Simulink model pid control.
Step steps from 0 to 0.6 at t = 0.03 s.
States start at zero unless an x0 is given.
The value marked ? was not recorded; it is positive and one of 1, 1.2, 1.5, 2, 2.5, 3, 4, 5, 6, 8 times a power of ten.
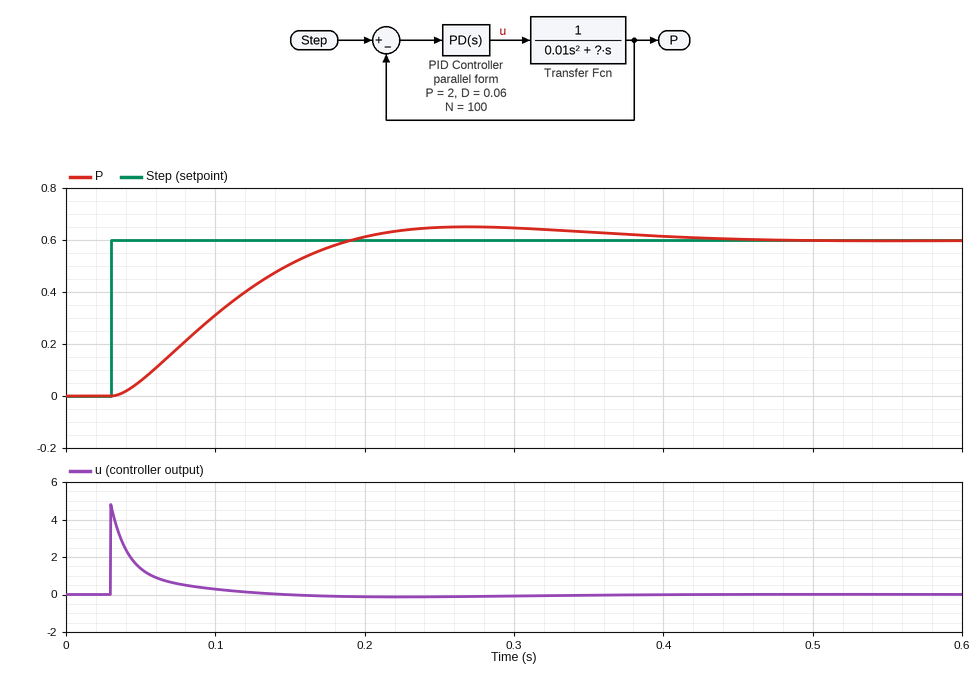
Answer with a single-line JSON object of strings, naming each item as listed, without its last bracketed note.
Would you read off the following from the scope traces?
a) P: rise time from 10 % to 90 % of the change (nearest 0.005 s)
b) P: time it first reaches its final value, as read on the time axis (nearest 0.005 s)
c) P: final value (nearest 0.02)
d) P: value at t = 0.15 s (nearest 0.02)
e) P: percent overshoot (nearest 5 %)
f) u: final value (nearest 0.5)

{"P: rise time from 10 % to 90 % of the change": "0.110 s", "P: time it first reaches its final value, as read on the time axis": "0.190 s", "P: final value": "0.60", "P: value at t = 0.15 s": "0.50", "P: percent overshoot": "10 %", "u: final value": "0.0"}
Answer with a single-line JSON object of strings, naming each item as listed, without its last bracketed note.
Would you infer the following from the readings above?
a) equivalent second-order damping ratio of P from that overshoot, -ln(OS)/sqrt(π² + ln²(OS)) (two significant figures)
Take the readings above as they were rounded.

{"equivalent second-order damping ratio of P from that overshoot, -ln(OS)/sqrt(π² + ln²(OS))": "0.59"}
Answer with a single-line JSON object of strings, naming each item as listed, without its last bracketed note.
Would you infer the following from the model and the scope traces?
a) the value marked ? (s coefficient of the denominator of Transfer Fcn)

{"the value marked ?": "0.12"}
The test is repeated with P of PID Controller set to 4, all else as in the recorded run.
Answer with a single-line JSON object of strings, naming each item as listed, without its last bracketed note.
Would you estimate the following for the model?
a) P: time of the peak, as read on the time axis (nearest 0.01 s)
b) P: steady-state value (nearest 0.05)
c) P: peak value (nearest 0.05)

{"P: time of the peak, as read on the time axis": "0.18 s", "P: steady-state value": "0.60", "P: peak value": "0.75"}
